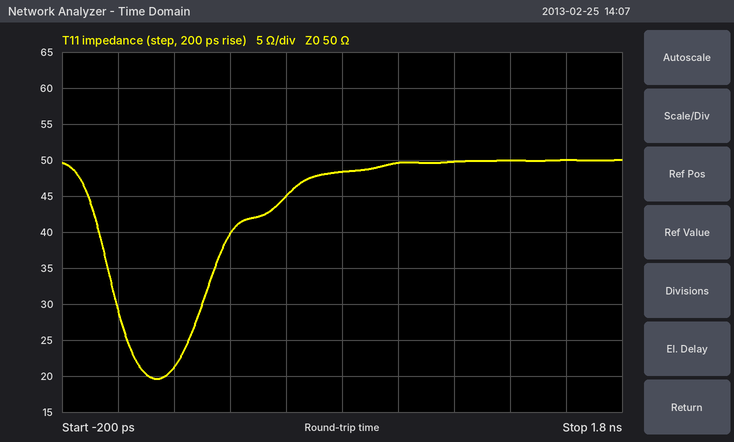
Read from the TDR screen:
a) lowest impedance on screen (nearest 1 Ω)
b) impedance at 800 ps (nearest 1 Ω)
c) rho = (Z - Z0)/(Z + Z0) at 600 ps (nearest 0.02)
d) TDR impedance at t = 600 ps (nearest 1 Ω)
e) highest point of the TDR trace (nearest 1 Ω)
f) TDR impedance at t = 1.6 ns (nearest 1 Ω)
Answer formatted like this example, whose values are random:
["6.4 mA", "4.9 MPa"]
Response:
["20 Ω", "48 Ω", "-0.06", "45 Ω", "50 Ω", "50 Ω"]
